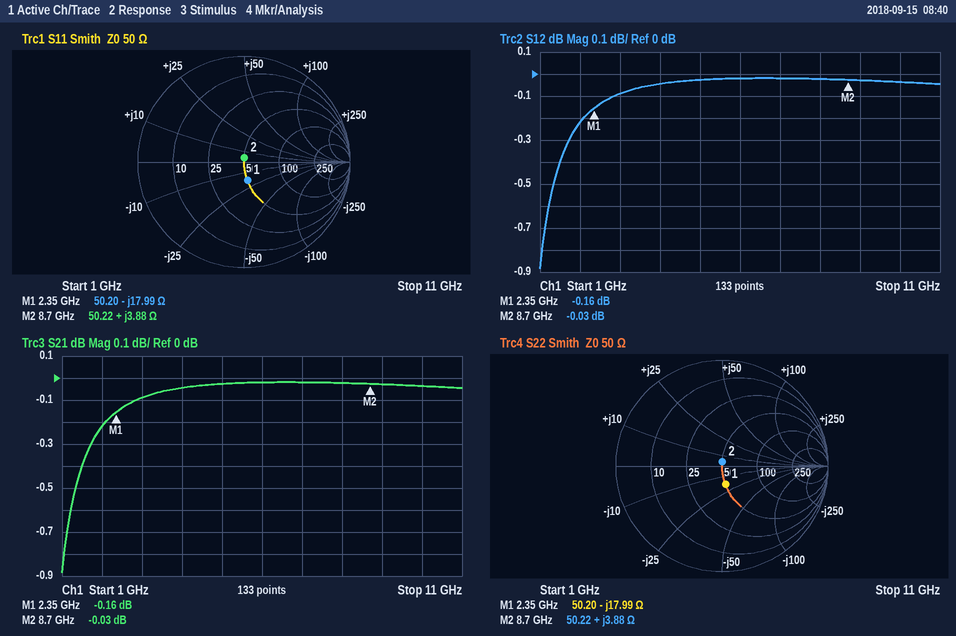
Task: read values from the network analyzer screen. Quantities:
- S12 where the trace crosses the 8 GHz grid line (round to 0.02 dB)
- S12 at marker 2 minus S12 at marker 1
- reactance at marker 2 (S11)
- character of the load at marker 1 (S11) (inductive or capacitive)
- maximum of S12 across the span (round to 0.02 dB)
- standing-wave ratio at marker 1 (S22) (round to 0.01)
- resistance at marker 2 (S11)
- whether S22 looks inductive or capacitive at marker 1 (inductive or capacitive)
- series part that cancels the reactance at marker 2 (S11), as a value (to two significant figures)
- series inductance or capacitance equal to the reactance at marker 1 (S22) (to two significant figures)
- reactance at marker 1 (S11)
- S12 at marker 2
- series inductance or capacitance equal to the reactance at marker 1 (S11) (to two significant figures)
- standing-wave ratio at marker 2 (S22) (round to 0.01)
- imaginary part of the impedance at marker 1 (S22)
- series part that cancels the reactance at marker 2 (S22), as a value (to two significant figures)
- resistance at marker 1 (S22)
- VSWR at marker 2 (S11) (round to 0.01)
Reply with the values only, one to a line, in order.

-0.02 dB
0.13 dB
+3.88 Ω
capacitive
-0.02 dB
1.43
50.22 Ω
capacitive
4.7 pF
3.8 pF
-17.99 Ω
-0.03 dB
3.8 pF
1.08
-17.99 Ω
4.7 pF
50.20 Ω
1.08
